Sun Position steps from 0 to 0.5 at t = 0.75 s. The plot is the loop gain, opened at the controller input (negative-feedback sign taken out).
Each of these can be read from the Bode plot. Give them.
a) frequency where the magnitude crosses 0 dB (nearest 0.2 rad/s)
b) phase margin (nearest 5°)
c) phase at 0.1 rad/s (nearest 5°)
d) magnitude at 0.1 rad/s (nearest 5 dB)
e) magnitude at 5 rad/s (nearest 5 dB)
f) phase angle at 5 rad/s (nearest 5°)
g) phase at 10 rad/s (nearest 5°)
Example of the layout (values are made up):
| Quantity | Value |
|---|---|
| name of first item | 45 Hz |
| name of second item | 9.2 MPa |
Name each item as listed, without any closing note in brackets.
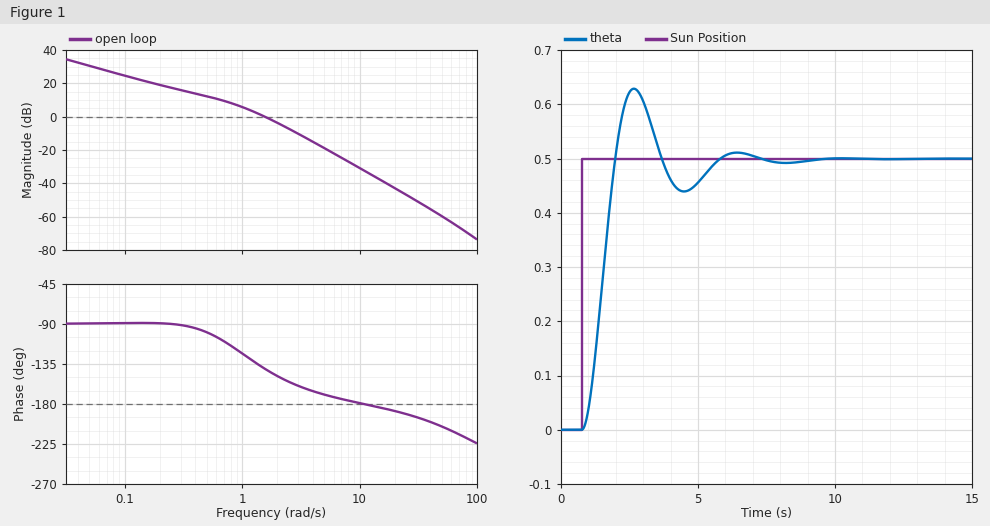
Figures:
| Quantity | Value |
|---|---|
| frequency where the magnitude crosses 0 dB | 1.6 rad/s |
| phase margin | 40° |
| phase at 0.1 rad/s | -90° |
| magnitude at 0.1 rad/s | 25 dB |
| magnitude at 5 rad/s | -20 dB |
| phase angle at 5 rad/s | -170° |
| phase at 10 rad/s | -180° |
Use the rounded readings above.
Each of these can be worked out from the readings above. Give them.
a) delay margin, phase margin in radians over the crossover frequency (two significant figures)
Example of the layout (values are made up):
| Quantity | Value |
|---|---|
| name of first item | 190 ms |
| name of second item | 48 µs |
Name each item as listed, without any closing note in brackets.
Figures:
| Quantity | Value |
|---|---|
| delay margin, phase margin in radians over the crossover frequency | 0.44 s |
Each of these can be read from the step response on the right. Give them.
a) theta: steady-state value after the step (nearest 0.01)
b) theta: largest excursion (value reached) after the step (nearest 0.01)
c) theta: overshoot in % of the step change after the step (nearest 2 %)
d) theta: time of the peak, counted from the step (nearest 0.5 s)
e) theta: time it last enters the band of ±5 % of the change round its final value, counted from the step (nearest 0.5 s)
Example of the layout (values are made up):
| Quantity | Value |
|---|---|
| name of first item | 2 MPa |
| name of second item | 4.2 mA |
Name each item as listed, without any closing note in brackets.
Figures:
| Quantity | Value |
|---|---|
| theta: steady-state value after the step | 0.50 |
| theta: largest excursion (value reached) after the step | 0.63 |
| theta: overshoot in % of the step change after the step | 26 % |
| theta: time of the peak, counted from the step | 2.0 s |
| theta: time it last enters the band of ±5 % of the change round its final value, counted from the step | 4.5 s |
